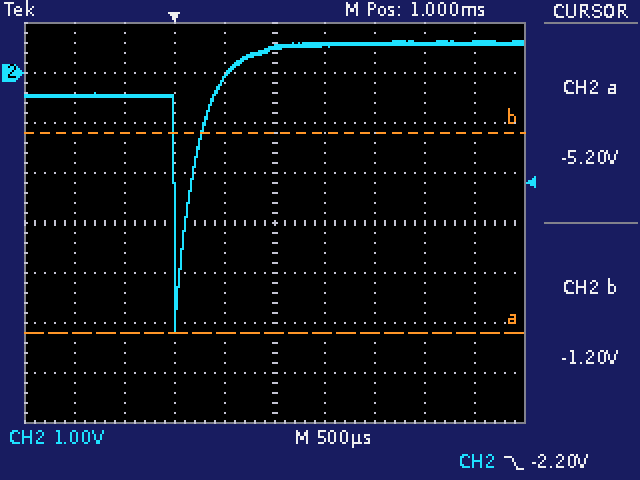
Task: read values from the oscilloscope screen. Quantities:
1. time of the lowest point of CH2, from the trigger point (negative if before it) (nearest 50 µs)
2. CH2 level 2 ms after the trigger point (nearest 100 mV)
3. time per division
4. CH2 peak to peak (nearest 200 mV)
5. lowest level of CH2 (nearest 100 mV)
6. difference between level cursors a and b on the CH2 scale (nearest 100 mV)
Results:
0 µs
600 mV
500 µs
5.8 V
-5.2 V
4.0 V
